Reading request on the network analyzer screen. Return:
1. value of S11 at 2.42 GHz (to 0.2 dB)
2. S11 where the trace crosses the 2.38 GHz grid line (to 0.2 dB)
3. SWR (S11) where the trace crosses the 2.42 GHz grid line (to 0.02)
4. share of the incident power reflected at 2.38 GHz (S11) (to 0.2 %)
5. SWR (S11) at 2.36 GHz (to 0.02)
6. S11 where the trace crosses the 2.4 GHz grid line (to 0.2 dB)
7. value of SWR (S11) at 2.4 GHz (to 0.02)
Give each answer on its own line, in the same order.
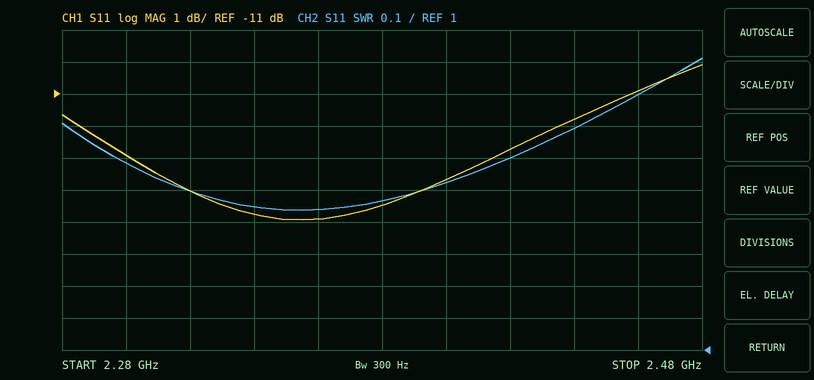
-12.8 dB
-14.4 dB
1.60
3.6 %
1.44
-13.6 dB
1.52
